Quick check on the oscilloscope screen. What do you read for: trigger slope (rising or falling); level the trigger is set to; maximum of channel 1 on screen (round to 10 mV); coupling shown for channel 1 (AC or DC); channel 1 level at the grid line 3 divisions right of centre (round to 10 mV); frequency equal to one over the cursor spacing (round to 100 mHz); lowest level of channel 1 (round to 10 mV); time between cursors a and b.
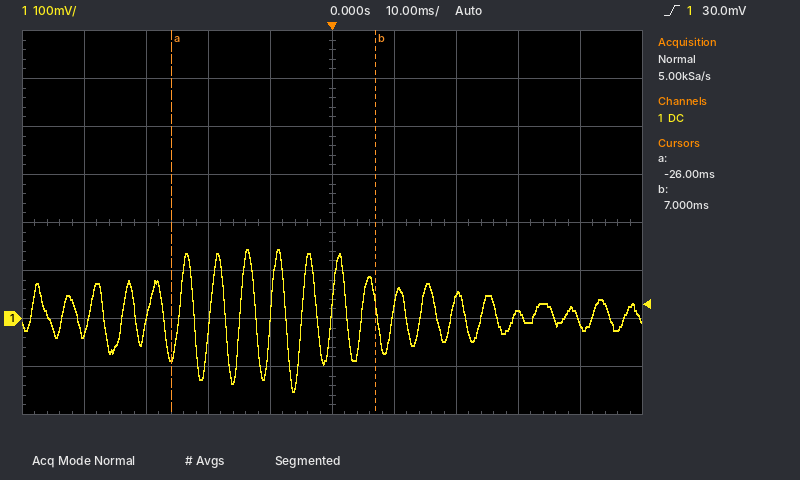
rising
30.0 mV
140 mV
DC
10 mV
30.3 Hz
-150 mV
33 ms
